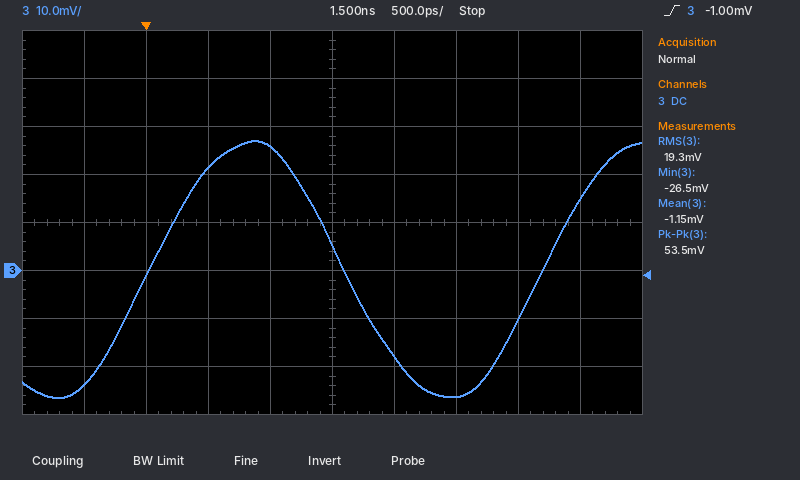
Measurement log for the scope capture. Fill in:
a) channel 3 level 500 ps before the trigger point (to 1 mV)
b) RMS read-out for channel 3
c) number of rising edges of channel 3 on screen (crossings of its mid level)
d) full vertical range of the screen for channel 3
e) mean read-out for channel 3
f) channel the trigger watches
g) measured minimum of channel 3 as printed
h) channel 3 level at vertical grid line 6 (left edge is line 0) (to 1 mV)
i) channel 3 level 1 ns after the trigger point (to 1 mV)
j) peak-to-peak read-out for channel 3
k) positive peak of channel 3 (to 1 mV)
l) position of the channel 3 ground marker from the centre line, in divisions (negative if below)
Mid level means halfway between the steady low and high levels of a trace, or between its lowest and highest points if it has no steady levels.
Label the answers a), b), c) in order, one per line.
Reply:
a) -24 mV
b) 19.3 mV
c) 2
d) 80 mV
e) -1.15 mV
f) channel 3
g) -26.5 mV
h) -18 mV
i) 26 mV
j) 53.5 mV
k) 27 mV
l) -1.0 div
